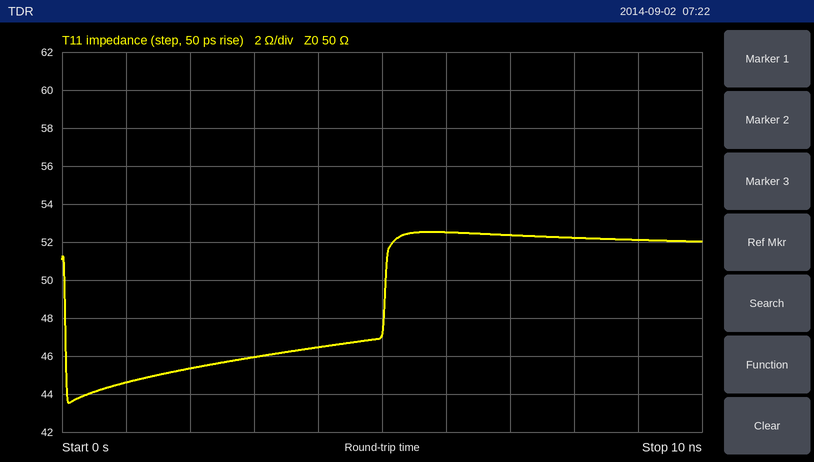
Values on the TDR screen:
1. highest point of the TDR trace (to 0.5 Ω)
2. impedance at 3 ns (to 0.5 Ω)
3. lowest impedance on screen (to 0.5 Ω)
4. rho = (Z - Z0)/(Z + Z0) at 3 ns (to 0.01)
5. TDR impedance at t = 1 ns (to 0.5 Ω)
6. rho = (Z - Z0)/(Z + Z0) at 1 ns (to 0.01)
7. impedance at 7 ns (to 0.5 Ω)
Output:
52.5 Ω
46.0 Ω
43.5 Ω
-0.04
44.5 Ω
-0.06
52.5 Ω
